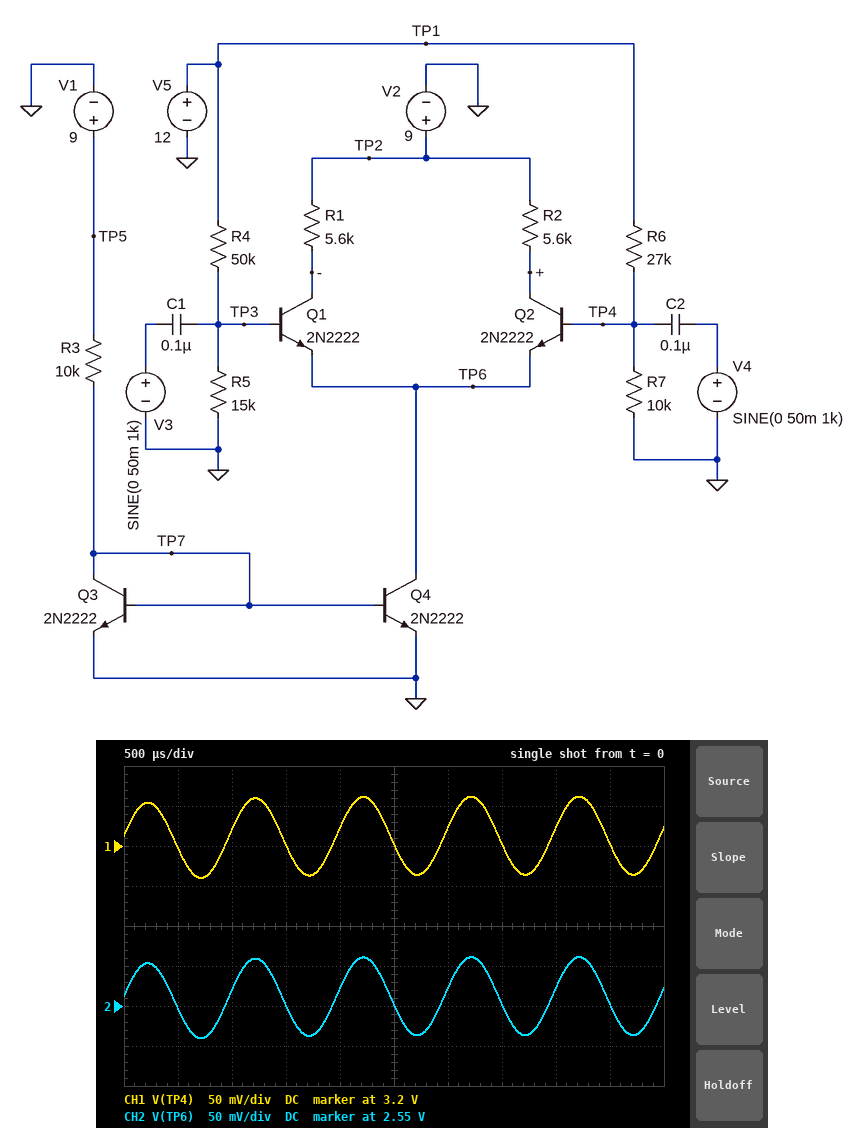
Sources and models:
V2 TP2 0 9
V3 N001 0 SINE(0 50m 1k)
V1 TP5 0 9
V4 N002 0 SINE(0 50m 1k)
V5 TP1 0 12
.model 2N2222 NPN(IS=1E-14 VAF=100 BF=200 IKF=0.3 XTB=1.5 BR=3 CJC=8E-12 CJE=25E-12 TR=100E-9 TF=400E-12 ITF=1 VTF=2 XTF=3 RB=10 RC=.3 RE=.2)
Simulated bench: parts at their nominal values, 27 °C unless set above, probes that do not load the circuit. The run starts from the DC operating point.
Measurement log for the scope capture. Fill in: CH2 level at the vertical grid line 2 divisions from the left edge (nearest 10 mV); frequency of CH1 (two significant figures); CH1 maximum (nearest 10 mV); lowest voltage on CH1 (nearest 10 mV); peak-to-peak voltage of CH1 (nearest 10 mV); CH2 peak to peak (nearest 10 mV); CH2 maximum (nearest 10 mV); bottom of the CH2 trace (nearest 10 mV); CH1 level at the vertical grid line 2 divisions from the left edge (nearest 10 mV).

2.57 V
1.0 kHz
3.26 V
3.16 V
100 mV
100 mV
2.61 V
2.51 V
3.22 V
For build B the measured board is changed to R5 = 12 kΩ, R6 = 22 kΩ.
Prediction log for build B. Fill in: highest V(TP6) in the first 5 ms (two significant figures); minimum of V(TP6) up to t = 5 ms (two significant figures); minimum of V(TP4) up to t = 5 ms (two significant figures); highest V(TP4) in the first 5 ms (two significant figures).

3.1 V
3.0 V
3.7 V
3.8 V
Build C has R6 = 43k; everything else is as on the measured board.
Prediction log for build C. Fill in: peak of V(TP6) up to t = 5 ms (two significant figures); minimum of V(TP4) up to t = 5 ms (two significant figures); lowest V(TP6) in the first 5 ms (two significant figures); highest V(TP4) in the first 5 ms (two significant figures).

2.1 V
2.2 V
2.0 V
2.3 V
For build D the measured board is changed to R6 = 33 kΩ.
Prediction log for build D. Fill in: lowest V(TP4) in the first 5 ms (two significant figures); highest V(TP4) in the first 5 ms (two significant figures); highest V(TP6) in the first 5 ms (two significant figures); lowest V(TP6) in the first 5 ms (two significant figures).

2.7 V
2.8 V
2.2 V
2.1 V
